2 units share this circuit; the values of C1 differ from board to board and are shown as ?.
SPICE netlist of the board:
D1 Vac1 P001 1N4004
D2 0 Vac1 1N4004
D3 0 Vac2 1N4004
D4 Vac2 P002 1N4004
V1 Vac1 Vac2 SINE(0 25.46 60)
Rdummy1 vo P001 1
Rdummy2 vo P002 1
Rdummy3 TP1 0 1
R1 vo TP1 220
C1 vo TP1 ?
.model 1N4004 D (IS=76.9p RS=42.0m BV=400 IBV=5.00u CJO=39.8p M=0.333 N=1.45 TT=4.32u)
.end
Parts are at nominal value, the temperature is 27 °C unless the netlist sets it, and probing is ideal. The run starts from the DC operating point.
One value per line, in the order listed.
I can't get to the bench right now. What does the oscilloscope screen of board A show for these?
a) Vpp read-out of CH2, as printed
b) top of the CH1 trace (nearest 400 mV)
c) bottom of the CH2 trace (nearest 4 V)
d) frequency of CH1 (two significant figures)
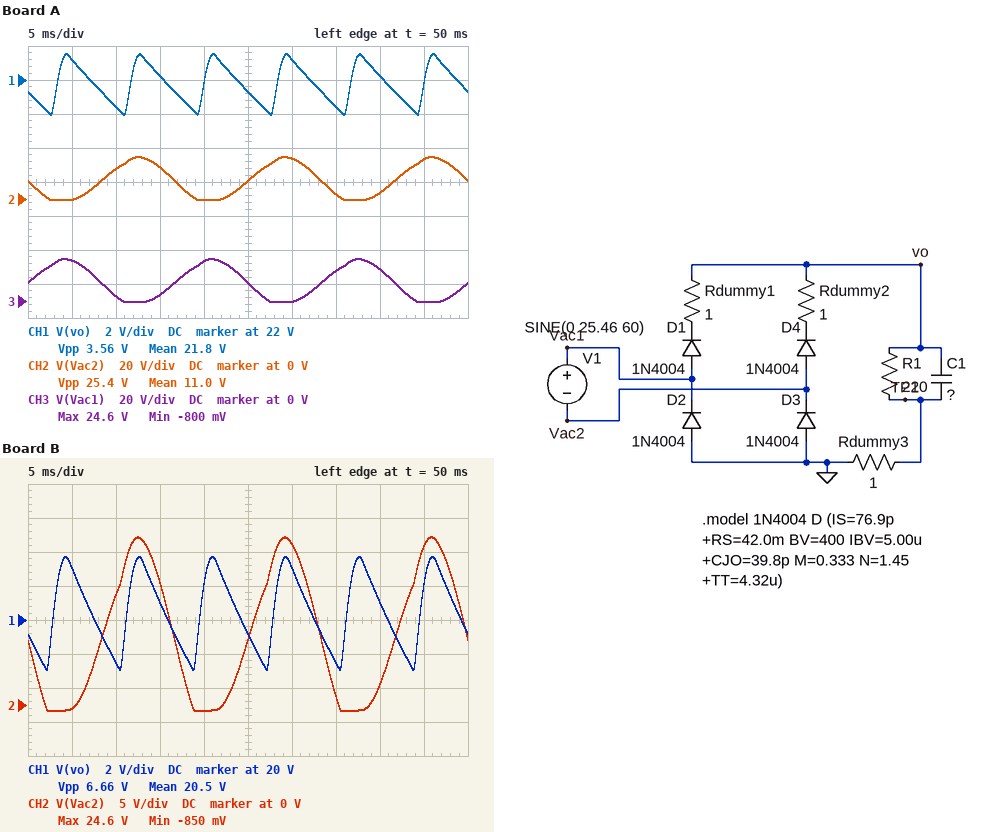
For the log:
25.4 V
23.6 V
0 V
120 Hz
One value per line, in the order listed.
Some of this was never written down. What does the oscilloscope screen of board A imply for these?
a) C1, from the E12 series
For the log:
180 µF
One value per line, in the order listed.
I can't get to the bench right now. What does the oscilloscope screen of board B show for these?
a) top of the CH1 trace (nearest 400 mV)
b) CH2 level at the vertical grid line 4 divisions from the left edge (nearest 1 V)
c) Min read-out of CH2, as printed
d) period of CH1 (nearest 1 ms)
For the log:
23.6 V
-1 V
-850 mV
8 ms
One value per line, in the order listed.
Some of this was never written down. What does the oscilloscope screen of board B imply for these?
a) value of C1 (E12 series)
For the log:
82 µF
